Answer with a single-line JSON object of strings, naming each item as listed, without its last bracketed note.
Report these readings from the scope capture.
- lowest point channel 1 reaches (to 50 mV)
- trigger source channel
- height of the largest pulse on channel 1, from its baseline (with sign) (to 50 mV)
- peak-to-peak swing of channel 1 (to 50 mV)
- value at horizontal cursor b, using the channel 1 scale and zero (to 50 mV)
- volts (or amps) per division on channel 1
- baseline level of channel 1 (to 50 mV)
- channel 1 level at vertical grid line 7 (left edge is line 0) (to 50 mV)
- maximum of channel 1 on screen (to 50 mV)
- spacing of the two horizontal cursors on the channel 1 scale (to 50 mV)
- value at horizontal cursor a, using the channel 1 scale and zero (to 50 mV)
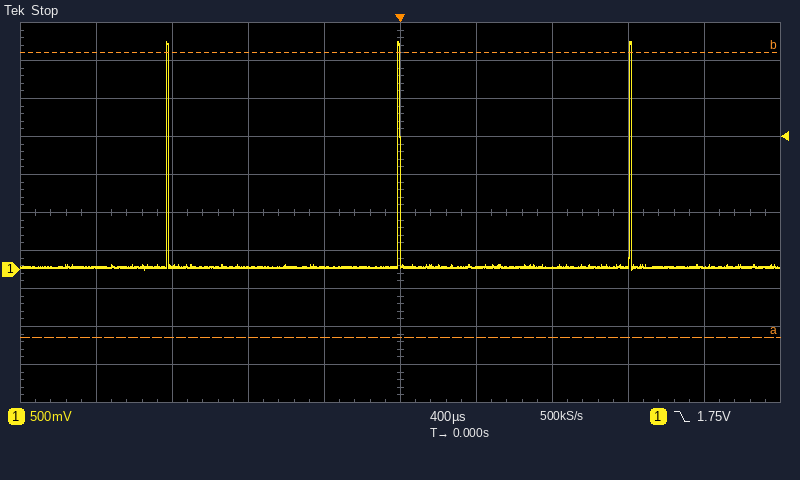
{"lowest point channel 1 reaches": "0 mV", "trigger source channel": "channel 1", "height of the largest pulse on channel 1, from its baseline (with sign)": "+2.95 V", "peak-to-peak swing of channel 1": "3.00 V", "value at horizontal cursor b, using the channel 1 scale and zero": "2.85 V", "volts (or amps) per division on channel 1": "500 mV", "baseline level of channel 1": "50 mV", "channel 1 level at vertical grid line 7 (left edge is line 0)": "50 mV", "maximum of channel 1 on screen": "3.00 V", "spacing of the two horizontal cursors on the channel 1 scale": "3.75 V", "value at horizontal cursor a, using the channel 1 scale and zero": "-900 mV"}
